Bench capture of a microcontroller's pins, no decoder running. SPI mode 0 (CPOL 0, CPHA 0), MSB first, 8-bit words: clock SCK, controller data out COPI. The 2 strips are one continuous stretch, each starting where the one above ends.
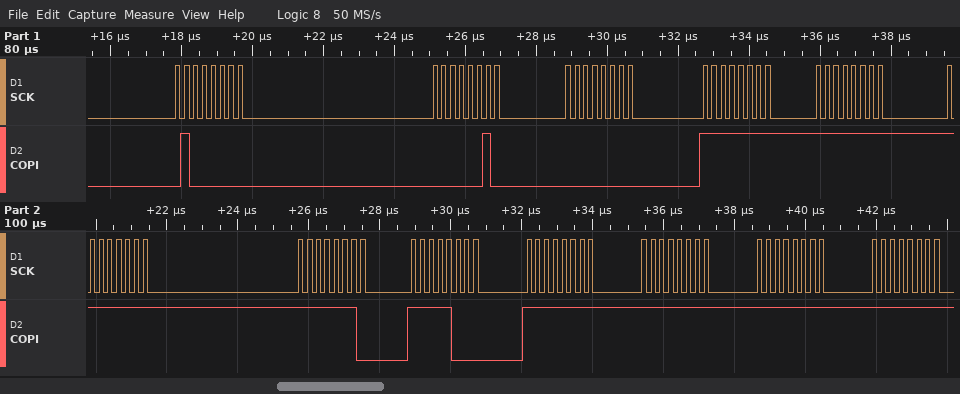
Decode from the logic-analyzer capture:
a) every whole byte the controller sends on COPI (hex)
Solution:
0x40 0x02 0x00 0xFF 0xFF 0xFF 0xFE 0xF8 0xFF 0xFF 0xFF 0xFF
